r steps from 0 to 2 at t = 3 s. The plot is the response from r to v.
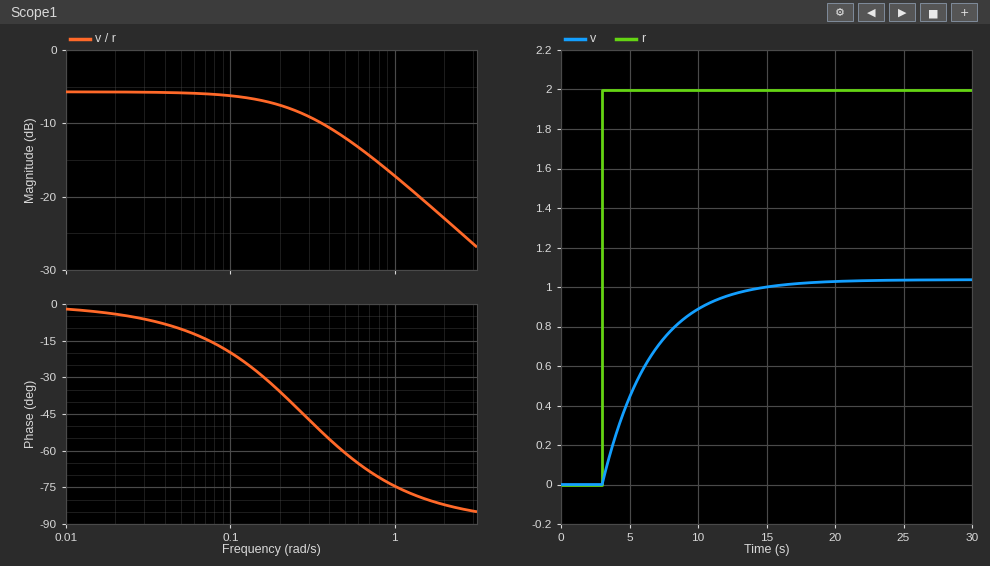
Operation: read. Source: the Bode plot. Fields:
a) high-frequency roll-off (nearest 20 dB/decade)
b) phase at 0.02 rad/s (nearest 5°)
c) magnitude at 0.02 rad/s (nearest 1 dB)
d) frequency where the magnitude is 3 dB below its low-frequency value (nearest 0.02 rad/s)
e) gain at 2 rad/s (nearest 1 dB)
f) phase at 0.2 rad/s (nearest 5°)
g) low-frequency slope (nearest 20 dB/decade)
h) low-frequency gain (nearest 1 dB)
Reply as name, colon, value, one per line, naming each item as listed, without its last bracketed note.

high-frequency roll-off: -20 dB/decade
phase at 0.02 rad/s: -5°
magnitude at 0.02 rad/s: -6 dB
frequency where the magnitude is 3 dB below its low-frequency value: 0.28 rad/s
gain at 2 rad/s: -23 dB
phase at 0.2 rad/s: -35°
low-frequency slope: 0 dB/decade
low-frequency gain: -6 dB
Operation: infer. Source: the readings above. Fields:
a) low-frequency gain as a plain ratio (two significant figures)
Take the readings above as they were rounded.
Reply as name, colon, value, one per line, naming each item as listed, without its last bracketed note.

low-frequency gain as a plain ratio: 0.50
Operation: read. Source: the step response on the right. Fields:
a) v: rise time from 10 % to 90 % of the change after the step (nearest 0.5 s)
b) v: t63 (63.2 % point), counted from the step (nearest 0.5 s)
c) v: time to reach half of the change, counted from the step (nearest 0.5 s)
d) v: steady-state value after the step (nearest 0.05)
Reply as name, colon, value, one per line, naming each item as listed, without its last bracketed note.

v: rise time from 10 % to 90 % of the change after the step: 8.0 s
v: t63 (63.2 % point), counted from the step: 3.5 s
v: time to reach half of the change, counted from the step: 2.5 s
v: steady-state value after the step: 1.05
